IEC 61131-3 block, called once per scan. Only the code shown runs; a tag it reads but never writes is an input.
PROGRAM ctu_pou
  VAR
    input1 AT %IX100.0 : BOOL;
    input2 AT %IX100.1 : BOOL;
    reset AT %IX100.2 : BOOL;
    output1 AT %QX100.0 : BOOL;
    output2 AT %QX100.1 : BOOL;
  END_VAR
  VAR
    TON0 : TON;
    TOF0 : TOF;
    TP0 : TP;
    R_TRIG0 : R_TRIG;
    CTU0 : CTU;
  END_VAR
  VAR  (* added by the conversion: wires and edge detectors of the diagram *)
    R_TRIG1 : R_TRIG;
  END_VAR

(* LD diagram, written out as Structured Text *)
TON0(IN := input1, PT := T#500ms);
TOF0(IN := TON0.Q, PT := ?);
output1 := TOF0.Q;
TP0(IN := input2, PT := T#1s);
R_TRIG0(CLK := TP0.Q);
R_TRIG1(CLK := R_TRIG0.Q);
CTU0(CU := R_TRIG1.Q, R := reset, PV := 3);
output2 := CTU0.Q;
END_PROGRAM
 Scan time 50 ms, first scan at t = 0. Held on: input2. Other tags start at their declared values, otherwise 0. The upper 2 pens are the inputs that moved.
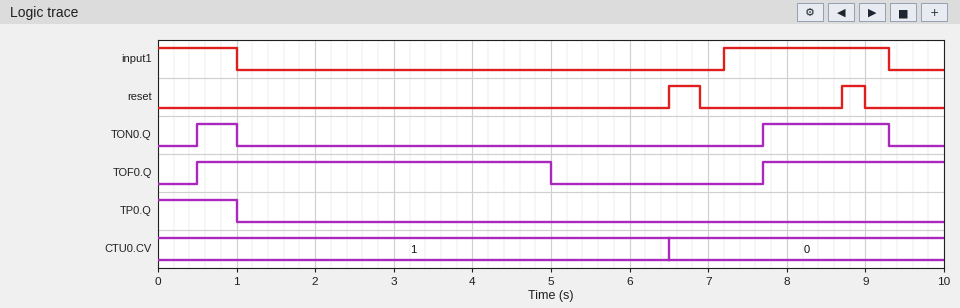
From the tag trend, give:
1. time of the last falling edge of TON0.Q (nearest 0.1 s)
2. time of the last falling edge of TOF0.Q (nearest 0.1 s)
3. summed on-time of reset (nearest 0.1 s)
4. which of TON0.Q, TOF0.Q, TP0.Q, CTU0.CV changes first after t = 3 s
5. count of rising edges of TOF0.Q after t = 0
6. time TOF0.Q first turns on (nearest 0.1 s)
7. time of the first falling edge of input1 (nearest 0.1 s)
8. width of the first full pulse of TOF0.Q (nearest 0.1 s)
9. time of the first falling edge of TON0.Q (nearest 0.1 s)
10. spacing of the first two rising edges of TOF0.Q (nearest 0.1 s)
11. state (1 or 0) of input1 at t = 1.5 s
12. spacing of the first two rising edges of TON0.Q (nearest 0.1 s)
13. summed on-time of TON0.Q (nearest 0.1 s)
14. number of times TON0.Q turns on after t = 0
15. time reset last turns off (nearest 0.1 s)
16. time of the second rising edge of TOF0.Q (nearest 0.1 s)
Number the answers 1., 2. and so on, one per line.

1. 9.3 s
2. 5.0 s
3. 0.7 s
4. TOF0.Q
5. 2
6. 0.5 s
7. 1.0 s
8. 4.5 s
9. 1.0 s
10. 7.2 s
11. 0
12. 7.2 s
13. 2.1 s
14. 2
15. 9.0 s
16. 7.7 s
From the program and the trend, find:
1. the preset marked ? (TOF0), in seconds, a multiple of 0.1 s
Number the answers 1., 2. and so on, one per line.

1. 4.0 s
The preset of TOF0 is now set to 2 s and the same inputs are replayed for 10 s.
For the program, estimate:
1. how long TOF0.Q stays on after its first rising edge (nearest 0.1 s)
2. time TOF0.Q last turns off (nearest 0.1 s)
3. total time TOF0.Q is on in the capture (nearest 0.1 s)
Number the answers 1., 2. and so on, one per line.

1. 2.5 s
2. 3.0 s
3. 4.8 s
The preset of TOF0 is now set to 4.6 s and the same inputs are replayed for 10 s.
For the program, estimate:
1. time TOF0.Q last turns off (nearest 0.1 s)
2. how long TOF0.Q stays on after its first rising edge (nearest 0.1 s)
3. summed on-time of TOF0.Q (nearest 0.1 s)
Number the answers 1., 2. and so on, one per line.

1. 5.6 s
2. 5.1 s
3. 7.4 s
